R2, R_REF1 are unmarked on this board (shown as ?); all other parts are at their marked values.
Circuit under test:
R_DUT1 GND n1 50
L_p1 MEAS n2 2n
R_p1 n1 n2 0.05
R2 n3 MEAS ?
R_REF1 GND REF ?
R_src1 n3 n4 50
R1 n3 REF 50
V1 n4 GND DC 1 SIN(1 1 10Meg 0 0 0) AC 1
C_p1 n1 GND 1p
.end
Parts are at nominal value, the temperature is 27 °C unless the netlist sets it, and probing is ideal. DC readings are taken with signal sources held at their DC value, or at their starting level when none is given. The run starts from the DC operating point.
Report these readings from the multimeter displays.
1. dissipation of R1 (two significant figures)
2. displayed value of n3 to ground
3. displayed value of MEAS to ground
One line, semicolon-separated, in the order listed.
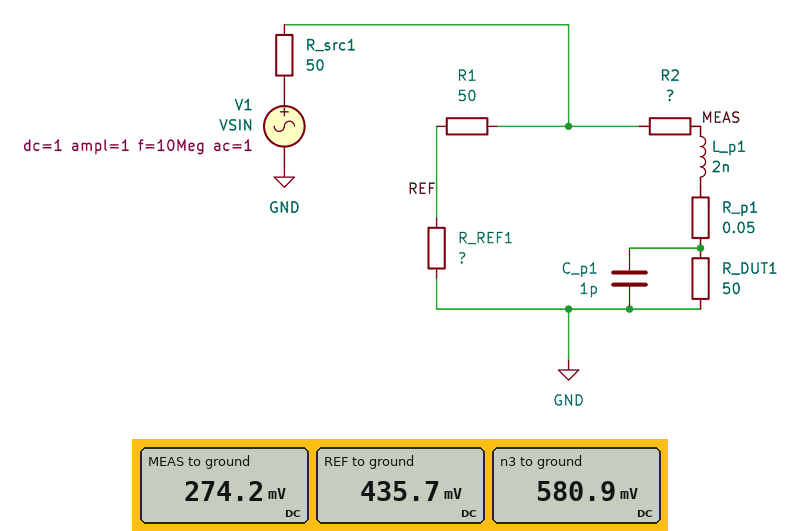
420 µW; 580.9 mV; 274.2 mV
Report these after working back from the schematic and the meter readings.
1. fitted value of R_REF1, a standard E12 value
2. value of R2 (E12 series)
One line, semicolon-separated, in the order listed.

150 Ω; 56 Ω
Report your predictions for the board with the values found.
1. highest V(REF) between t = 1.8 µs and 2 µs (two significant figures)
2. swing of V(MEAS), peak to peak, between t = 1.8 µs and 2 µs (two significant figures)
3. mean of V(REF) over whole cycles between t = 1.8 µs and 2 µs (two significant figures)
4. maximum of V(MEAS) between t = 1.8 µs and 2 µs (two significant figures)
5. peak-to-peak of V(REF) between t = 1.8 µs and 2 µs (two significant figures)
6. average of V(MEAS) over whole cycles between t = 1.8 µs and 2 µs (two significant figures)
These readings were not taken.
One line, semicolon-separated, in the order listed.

870 mV; 550 mV; 440 mV; 550 mV; 870 mV; 270 mV
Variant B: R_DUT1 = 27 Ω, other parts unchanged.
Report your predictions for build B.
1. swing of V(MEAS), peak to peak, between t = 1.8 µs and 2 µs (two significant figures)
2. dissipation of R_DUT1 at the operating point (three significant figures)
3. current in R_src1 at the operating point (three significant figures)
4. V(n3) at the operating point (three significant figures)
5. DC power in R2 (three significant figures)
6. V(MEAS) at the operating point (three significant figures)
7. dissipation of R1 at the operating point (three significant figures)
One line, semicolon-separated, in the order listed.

350 mV; 1.14 mW; 9.20 mA; 540 mV; 2.37 mW; 176 mV; 364 µW
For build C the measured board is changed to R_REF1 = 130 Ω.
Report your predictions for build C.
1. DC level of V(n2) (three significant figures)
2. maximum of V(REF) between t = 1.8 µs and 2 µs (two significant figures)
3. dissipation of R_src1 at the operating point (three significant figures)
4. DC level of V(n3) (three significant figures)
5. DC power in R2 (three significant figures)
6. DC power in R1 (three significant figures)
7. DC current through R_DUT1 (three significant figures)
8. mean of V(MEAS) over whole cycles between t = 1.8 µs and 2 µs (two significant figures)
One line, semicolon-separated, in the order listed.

270 mV; 830 mV; 3.67 mW; 572 mV; 1.63 mW; 504 µW; 5.39 mA; 270 mV
